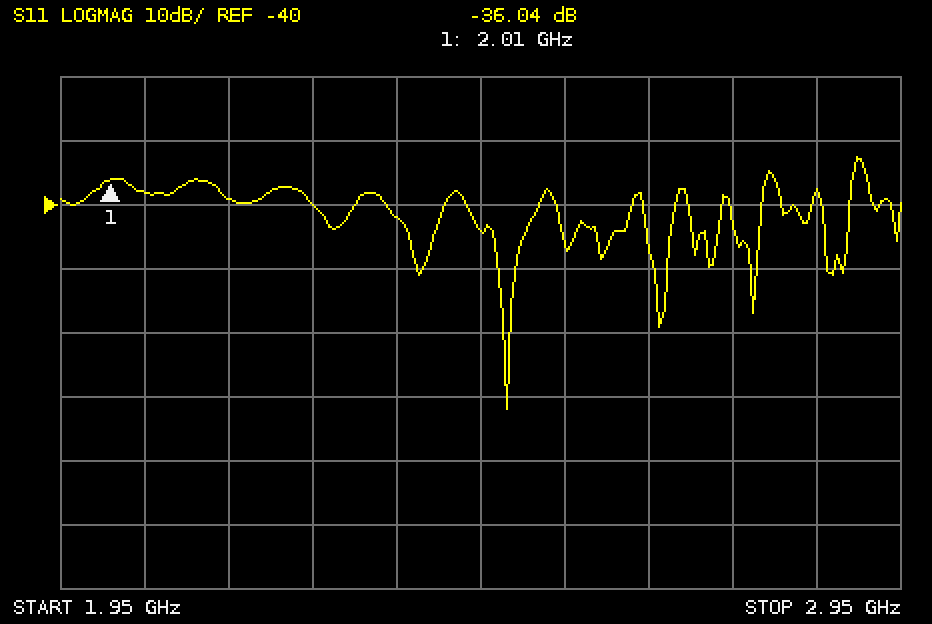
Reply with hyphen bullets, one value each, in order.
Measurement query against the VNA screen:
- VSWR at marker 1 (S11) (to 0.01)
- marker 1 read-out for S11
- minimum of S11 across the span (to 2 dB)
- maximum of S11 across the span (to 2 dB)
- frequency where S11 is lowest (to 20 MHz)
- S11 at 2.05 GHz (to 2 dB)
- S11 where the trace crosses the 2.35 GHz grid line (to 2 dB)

- 1.03
- -36.04 dB
- -72 dB
- -32 dB
- 2.48 GHz
- -38 dB
- -42 dB
